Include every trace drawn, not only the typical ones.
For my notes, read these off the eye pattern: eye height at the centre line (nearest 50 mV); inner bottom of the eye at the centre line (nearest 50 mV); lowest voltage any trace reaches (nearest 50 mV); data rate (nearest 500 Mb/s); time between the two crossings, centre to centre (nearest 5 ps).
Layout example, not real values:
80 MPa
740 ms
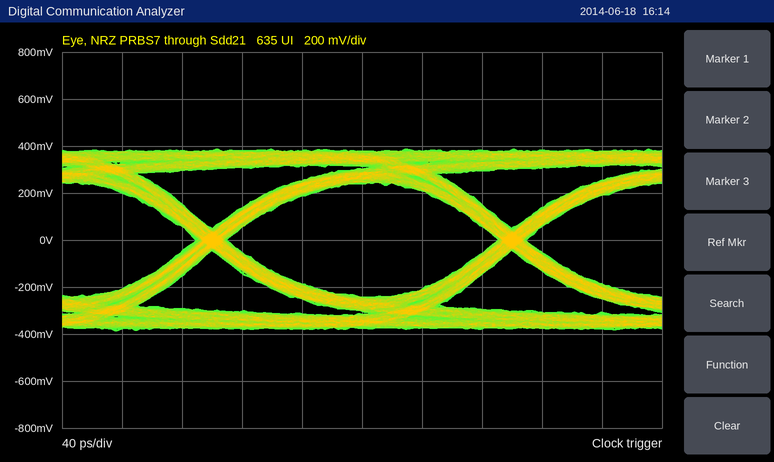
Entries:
500 mV
-250 mV
-400 mV
5.0 Gb/s
200 ps
